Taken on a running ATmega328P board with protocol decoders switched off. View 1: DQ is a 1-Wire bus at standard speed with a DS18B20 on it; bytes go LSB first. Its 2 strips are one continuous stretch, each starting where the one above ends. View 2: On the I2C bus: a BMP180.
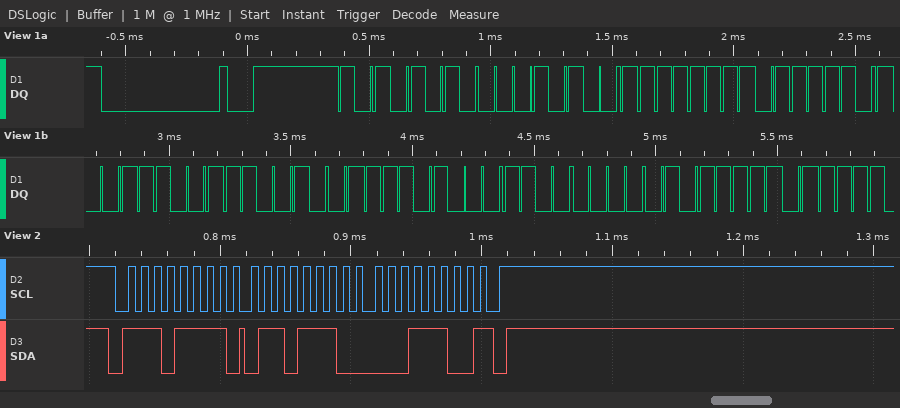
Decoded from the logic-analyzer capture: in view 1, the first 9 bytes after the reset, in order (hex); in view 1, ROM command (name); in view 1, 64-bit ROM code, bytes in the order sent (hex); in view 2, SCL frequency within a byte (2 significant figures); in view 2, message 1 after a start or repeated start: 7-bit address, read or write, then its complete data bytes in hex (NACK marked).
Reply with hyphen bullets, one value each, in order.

- 55 28 FF BE 9C 93 17 03 FA
- Match ROM
- 28 FF BE 9C 93 17 03 FA
- 100 kHz
- 0x77 read: 6E 1C NACK
